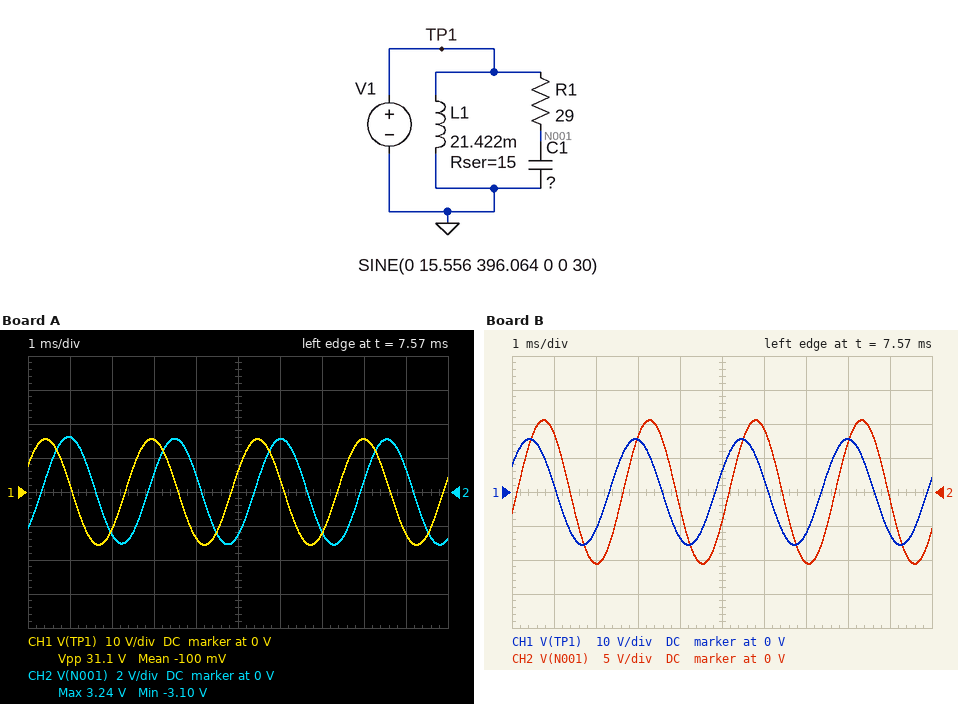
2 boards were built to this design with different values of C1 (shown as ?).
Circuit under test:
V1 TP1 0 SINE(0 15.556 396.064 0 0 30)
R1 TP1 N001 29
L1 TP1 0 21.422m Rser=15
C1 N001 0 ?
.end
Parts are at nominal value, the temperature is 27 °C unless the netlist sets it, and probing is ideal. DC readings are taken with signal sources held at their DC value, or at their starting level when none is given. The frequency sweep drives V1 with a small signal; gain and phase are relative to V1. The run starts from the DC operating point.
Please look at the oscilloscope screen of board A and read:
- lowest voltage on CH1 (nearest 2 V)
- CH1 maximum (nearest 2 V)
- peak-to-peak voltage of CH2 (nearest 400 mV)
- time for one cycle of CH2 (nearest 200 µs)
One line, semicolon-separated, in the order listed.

-16 V; 16 V; 6.4 V; 2.6 ms
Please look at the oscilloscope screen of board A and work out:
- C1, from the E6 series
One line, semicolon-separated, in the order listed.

68 µF
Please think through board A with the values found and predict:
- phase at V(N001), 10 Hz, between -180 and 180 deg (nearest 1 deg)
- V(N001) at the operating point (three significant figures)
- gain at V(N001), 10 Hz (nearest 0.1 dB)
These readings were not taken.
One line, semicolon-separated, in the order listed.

-7 deg; 7.78 V; -0.1 dB
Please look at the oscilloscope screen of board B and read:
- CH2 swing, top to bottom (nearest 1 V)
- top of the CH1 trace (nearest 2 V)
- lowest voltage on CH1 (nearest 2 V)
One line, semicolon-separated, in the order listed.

21 V; 16 V; -16 V
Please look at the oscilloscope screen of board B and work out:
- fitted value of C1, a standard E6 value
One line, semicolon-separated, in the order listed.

15 µF
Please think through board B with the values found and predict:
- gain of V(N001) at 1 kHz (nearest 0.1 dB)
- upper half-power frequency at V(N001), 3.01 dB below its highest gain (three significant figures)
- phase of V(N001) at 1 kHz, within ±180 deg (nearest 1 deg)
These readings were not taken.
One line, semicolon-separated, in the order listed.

-9.3 dB; 366 Hz; -70 deg
